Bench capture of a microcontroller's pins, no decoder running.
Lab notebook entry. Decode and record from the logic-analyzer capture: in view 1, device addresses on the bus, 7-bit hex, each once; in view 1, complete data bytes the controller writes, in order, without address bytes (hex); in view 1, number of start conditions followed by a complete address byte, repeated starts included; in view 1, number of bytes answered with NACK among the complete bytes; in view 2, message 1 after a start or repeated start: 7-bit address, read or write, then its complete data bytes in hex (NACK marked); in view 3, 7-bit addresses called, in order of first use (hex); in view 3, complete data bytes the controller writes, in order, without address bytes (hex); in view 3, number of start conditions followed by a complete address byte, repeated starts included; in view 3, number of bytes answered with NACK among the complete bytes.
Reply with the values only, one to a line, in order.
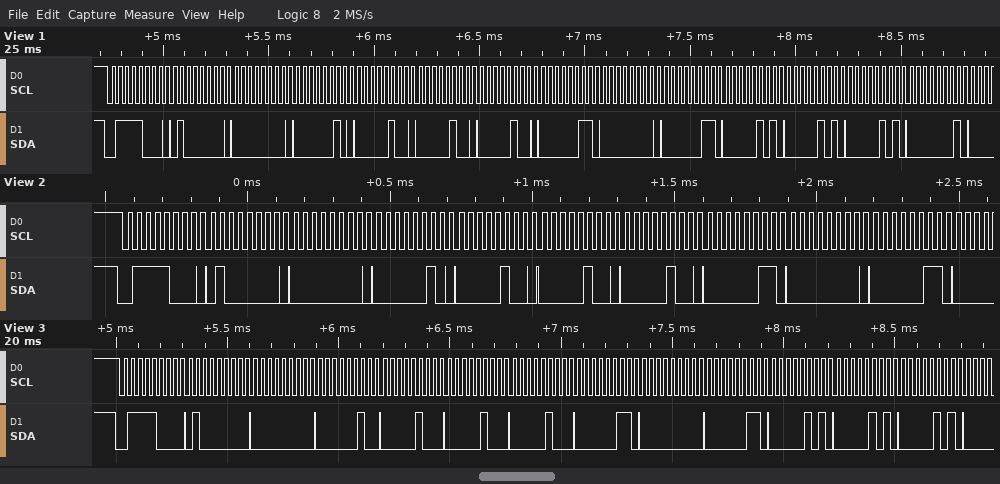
0x3C
40 00 02 04 04 04 03 00 03 05 05 05 01
1
0
0x3C write: 40 00 02 04 04 04 03 00 03
0x3C
40 00 02 04 04 04 03 00 03 05 05 05
1
0
